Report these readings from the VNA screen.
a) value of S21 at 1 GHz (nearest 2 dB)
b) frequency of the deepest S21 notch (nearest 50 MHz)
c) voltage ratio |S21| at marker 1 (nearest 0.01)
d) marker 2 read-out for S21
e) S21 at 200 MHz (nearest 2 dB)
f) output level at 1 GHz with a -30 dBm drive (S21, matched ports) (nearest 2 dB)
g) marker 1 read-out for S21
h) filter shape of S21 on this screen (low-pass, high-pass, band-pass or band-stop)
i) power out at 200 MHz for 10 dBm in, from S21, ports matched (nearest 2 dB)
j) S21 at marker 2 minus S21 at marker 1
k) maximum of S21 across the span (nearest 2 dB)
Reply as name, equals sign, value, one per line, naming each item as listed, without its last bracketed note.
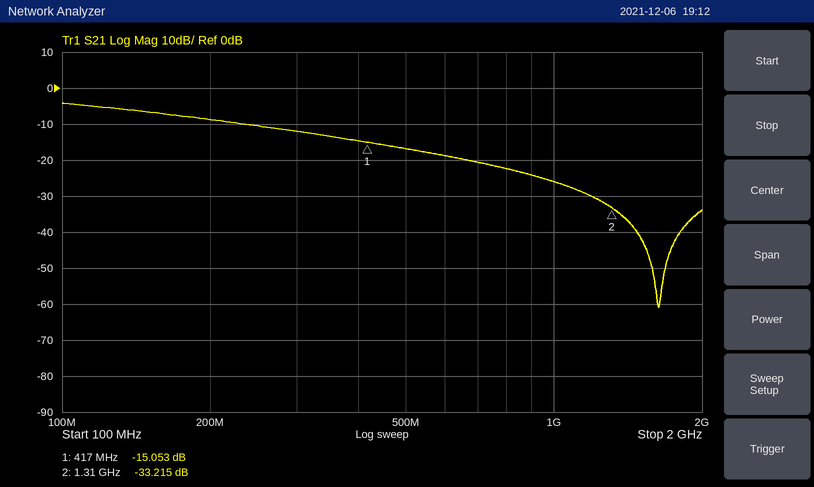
value of S21 at 1 GHz = -26 dB
frequency of the deepest S21 notch = 1.65 GHz
voltage ratio |S21| at marker 1 = 0.18
marker 2 read-out for S21 = -33.215 dB
S21 at 200 MHz = -8 dB
output level at 1 GHz with a -30 dBm drive (S21, matched ports) = -56 dBm
marker 1 read-out for S21 = -15.053 dB
filter shape of S21 on this screen = low-pass
power out at 200 MHz for 10 dBm in, from S21, ports matched = 2 dBm
S21 at marker 2 minus S21 at marker 1 = -18.162 dB
maximum of S21 across the span = -4 dB
